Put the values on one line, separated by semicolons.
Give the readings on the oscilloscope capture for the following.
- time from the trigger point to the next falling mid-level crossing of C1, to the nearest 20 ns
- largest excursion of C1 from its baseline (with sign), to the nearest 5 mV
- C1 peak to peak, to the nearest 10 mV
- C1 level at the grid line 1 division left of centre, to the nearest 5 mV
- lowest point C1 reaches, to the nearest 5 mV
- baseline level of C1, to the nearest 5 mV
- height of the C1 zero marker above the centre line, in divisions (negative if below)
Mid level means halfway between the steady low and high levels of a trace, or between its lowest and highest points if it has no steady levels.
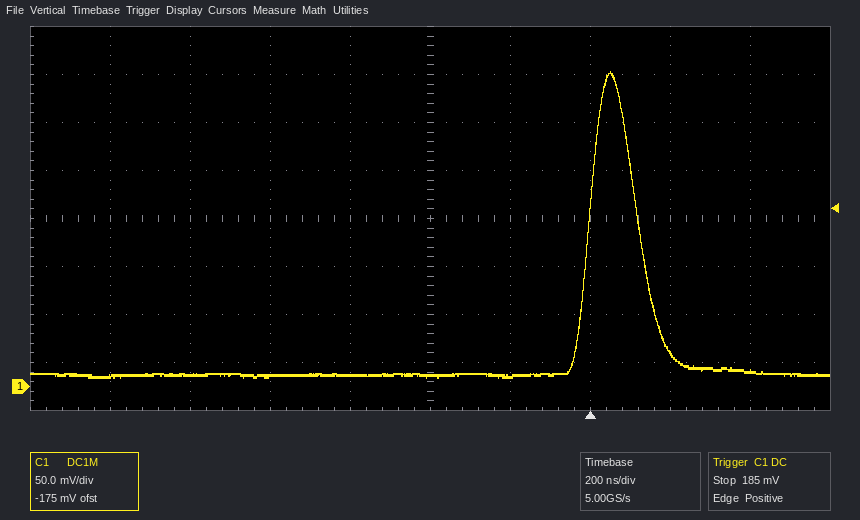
120 ns; +315 mV; 320 mV; 10 mV; 10 mV; 10 mV; -3.5 div
